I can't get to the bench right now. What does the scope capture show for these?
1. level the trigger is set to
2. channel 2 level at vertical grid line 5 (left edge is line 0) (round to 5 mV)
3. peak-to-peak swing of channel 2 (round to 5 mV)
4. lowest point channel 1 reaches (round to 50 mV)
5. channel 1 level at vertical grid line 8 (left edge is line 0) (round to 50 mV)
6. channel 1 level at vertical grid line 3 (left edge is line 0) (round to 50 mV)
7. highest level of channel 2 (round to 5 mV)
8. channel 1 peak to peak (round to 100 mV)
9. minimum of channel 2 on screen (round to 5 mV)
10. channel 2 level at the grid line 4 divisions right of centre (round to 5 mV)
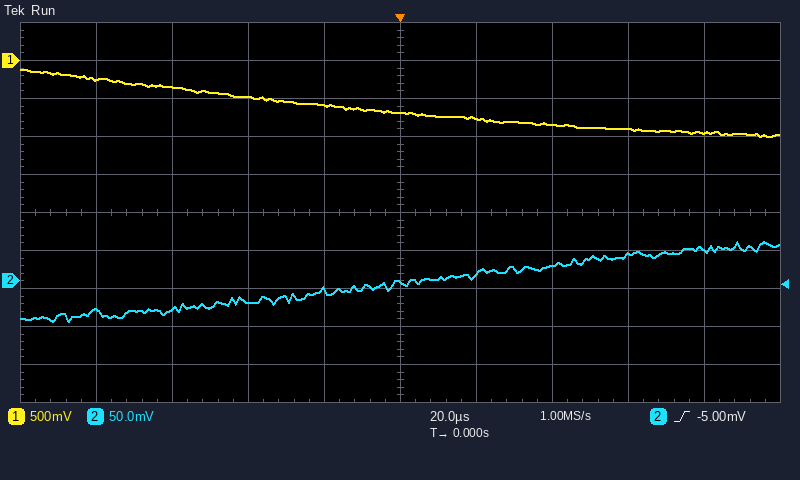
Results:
-5.00 mV
0 mV
105 mV
-1.00 V
-900 mV
-500 mV
50 mV
900 mV
-55 mV
40 mV
